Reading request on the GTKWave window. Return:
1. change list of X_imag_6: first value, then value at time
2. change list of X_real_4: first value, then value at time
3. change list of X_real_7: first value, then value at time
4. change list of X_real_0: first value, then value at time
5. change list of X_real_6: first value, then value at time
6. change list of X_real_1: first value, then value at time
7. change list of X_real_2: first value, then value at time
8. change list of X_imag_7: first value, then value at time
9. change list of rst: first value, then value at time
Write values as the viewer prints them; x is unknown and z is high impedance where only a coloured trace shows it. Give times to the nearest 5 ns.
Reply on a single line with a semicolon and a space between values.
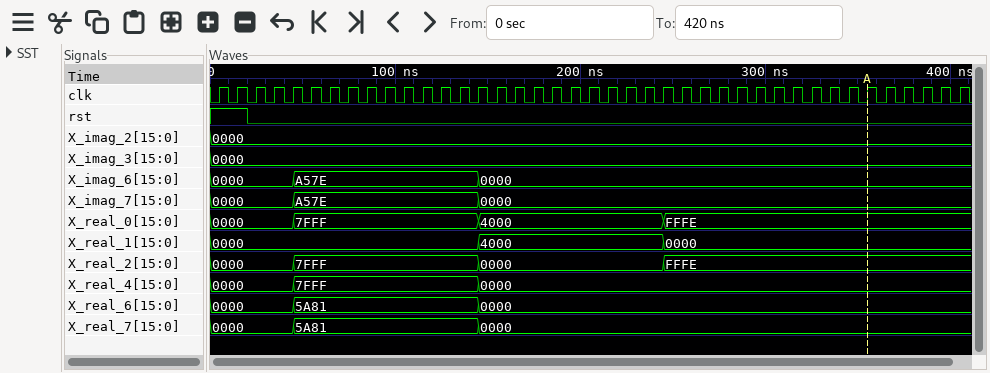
0000, A57E at 45 ns, 0000 at 145 ns; 0000, 7FFF at 45 ns, 0000 at 145 ns; 0000, 5A81 at 45 ns, 0000 at 145 ns; 0000, 7FFF at 45 ns, 4000 at 145 ns, FFFE at 245 ns; 0000, 5A81 at 45 ns, 0000 at 145 ns; 0000, 4000 at 145 ns, 0000 at 245 ns; 0000, 7FFF at 45 ns, 0000 at 145 ns, FFFE at 245 ns; 0000, A57E at 45 ns, 0000 at 145 ns; 1, 0 at 20 ns
